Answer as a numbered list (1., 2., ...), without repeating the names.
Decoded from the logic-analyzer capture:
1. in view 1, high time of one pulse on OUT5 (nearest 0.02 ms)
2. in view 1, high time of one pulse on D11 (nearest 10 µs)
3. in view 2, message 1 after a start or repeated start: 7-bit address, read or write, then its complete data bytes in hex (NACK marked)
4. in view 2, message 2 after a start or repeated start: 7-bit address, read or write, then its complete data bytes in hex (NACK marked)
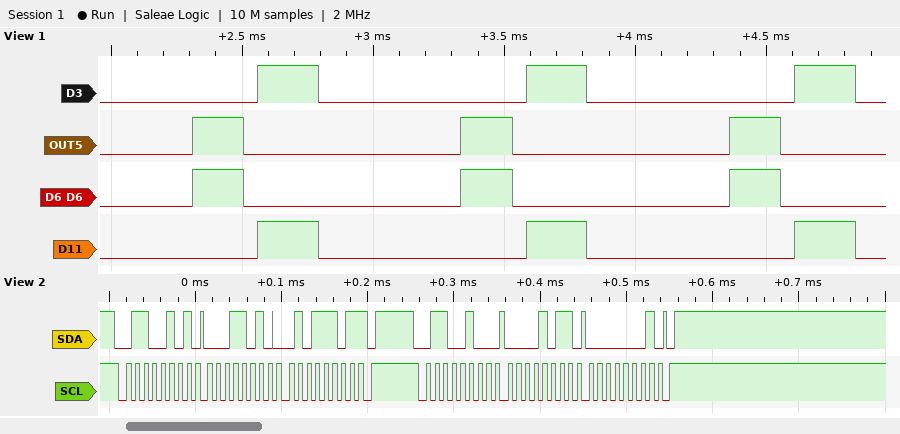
1. 0.20 ms
2. 230 µs
3. 0x32 read: 1A 5D NACK
4. 0x32 write: 0B 01
